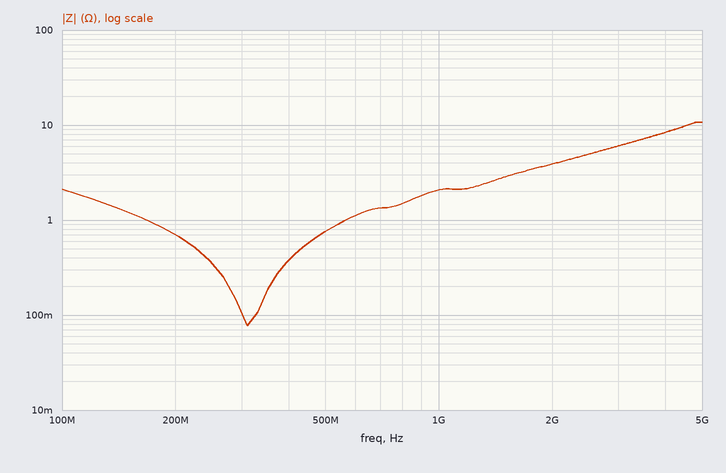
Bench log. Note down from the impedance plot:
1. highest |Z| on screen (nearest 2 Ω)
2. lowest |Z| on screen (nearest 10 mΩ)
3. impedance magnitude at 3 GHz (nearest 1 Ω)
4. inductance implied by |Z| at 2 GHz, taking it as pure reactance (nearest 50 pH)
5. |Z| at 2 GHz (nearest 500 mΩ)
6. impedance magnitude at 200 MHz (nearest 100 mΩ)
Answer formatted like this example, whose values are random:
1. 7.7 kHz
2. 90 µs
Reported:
1. 10 Ω
2. 80 mΩ
3. 6 Ω
4. 300 pH
5. 4.0 Ω
6. 700 mΩ
